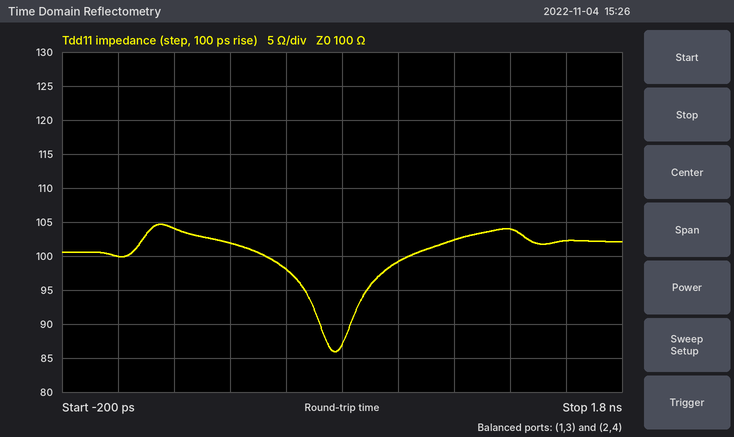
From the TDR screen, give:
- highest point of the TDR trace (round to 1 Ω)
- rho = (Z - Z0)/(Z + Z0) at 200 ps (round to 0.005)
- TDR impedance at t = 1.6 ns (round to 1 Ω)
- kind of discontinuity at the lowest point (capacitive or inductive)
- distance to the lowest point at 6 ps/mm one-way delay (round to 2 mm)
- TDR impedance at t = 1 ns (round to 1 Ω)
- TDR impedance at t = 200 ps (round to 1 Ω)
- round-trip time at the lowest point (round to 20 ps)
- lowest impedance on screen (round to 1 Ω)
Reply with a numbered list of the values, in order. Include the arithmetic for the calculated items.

1. 105 Ω
2. (104 − 100)/(104 + 100) ≈ +0.020
3. 102 Ω
4. capacitive
5. 780 ps / 2 / 6 ps/mm ≈ 65.0 mm, so 64 mm to the nearest 2 mm
6. 99 Ω
7. 104 Ω
8. 780 ps
9. 86 Ω
